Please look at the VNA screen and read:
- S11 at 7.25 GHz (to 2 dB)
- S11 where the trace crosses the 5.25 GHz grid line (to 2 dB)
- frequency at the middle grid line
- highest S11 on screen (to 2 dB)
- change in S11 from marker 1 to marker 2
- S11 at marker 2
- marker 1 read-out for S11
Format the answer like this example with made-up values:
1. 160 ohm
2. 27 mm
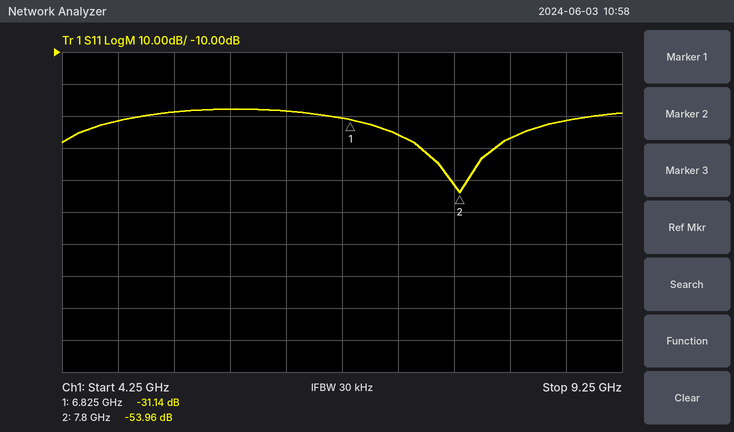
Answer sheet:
1. -36 dB
2. -28 dB
3. 6.75 GHz
4. -28 dB
5. -22.82 dB
6. -53.96 dB
7. -31.14 dB
